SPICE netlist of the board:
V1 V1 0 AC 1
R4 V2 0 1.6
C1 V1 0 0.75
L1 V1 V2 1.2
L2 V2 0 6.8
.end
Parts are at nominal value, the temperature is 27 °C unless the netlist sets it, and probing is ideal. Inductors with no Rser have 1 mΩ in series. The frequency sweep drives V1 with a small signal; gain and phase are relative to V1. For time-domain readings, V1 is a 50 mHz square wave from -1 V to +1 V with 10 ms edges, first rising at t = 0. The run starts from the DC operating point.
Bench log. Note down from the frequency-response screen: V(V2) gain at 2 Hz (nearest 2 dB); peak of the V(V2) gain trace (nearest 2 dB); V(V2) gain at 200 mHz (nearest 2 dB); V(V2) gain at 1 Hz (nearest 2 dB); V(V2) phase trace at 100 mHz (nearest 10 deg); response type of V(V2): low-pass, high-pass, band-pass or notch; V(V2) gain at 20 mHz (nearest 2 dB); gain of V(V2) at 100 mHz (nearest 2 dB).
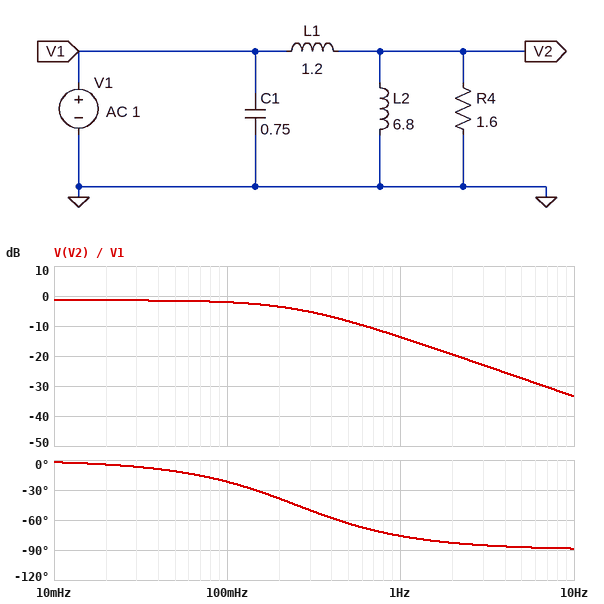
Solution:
-20 dB
-2 dB
-4 dB
-14 dB
-20 deg
low-pass
-2 dB
-2 dB
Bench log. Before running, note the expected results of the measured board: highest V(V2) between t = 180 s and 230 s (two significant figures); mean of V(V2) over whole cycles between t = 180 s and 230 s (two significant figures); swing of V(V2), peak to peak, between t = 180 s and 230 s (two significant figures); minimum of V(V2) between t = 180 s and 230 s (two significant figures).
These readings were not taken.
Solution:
1.2 V
330 mV
1.7 V
-520 mV
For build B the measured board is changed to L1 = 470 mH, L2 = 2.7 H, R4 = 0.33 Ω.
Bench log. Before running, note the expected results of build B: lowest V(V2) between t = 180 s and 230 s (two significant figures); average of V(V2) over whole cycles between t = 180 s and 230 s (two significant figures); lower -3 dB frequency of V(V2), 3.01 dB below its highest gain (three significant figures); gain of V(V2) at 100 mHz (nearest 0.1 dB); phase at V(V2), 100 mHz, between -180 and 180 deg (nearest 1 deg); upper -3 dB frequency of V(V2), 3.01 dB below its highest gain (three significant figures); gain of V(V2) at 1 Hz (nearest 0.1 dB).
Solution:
-540 mV
310 mV
55.7 µHz
-3.4 dB
-37 deg
132 mHz
-19.1 dB
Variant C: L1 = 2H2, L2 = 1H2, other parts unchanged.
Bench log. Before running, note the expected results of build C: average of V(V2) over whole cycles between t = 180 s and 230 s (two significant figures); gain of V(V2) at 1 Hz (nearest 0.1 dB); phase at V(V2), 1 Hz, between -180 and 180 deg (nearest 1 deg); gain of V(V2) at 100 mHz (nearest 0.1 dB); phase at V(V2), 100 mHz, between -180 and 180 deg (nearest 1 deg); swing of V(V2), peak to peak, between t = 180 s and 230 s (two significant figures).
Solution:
-130 mV
-19.2 dB
-72 deg
-9.4 dB
-17 deg
710 mV
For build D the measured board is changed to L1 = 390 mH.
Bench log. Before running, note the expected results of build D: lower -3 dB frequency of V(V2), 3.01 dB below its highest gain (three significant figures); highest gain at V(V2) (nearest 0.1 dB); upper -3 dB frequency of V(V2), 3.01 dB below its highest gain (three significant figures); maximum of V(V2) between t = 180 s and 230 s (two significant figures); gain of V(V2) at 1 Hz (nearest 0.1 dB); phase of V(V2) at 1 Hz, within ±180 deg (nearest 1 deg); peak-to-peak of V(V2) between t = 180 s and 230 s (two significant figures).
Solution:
29.4 µHz
-0.5 dB
691 mHz
1.4 V
-5.4 dB
-55 deg
1.9 V
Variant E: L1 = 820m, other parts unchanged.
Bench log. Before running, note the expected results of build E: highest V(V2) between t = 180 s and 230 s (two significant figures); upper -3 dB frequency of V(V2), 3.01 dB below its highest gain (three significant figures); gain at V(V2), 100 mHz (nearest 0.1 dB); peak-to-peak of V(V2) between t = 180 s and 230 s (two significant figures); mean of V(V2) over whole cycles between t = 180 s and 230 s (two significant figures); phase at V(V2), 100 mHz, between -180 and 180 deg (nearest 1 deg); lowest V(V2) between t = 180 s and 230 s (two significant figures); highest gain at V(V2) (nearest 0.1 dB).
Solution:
1.3 V
348 mHz
-1.3 dB
1.8 V
370 mV
-16 deg
-520 mV
-1.0 dB
